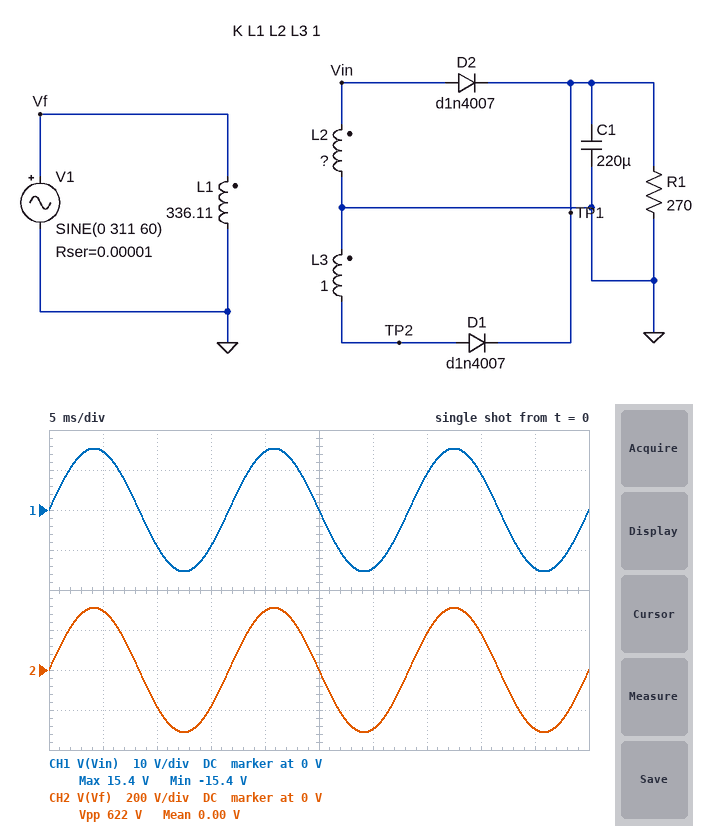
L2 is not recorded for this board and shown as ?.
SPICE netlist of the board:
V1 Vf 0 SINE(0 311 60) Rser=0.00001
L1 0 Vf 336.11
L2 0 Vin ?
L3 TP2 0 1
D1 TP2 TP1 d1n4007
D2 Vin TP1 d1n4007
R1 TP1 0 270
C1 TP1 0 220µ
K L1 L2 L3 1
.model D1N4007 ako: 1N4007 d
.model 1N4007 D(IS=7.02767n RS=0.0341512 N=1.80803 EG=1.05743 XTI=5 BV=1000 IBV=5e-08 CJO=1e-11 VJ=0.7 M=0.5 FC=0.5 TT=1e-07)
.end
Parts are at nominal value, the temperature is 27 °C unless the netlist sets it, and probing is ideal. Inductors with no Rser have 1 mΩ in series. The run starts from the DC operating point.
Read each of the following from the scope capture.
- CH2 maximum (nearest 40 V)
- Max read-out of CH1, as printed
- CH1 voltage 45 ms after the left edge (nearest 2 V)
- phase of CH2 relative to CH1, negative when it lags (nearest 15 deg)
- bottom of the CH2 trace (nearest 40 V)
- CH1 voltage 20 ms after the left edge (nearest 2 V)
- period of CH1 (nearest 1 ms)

320 V
15.4 V
-14 V
0 deg
-320 V
14 V
17 ms
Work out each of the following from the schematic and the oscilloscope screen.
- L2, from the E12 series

820 mH
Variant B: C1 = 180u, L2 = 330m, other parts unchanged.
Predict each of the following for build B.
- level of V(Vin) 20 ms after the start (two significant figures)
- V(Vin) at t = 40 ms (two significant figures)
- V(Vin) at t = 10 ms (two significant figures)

9.3 V
5.7 V
-5.7 V
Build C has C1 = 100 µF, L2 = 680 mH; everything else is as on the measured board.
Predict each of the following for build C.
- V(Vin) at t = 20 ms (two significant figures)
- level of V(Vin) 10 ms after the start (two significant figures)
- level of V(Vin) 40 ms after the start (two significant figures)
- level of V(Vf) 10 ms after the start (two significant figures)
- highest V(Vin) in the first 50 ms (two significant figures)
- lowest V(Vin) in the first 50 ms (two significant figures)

13 V
-8.2 V
8.2 V
-180 V
14 V
-14 V
